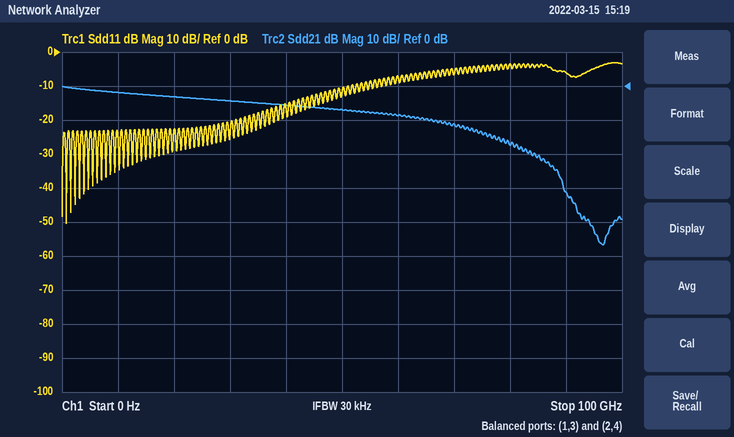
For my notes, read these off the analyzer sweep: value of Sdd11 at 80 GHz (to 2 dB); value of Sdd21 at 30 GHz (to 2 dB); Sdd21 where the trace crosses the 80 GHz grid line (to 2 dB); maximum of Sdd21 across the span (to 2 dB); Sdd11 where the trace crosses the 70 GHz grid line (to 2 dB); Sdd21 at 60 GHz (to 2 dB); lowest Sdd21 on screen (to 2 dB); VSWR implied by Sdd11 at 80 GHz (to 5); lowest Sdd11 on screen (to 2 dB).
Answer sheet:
-4 dB
-4 dB
-18 dB
0 dB
-6 dB
-8 dB
-46 dB
5
-50 dB
